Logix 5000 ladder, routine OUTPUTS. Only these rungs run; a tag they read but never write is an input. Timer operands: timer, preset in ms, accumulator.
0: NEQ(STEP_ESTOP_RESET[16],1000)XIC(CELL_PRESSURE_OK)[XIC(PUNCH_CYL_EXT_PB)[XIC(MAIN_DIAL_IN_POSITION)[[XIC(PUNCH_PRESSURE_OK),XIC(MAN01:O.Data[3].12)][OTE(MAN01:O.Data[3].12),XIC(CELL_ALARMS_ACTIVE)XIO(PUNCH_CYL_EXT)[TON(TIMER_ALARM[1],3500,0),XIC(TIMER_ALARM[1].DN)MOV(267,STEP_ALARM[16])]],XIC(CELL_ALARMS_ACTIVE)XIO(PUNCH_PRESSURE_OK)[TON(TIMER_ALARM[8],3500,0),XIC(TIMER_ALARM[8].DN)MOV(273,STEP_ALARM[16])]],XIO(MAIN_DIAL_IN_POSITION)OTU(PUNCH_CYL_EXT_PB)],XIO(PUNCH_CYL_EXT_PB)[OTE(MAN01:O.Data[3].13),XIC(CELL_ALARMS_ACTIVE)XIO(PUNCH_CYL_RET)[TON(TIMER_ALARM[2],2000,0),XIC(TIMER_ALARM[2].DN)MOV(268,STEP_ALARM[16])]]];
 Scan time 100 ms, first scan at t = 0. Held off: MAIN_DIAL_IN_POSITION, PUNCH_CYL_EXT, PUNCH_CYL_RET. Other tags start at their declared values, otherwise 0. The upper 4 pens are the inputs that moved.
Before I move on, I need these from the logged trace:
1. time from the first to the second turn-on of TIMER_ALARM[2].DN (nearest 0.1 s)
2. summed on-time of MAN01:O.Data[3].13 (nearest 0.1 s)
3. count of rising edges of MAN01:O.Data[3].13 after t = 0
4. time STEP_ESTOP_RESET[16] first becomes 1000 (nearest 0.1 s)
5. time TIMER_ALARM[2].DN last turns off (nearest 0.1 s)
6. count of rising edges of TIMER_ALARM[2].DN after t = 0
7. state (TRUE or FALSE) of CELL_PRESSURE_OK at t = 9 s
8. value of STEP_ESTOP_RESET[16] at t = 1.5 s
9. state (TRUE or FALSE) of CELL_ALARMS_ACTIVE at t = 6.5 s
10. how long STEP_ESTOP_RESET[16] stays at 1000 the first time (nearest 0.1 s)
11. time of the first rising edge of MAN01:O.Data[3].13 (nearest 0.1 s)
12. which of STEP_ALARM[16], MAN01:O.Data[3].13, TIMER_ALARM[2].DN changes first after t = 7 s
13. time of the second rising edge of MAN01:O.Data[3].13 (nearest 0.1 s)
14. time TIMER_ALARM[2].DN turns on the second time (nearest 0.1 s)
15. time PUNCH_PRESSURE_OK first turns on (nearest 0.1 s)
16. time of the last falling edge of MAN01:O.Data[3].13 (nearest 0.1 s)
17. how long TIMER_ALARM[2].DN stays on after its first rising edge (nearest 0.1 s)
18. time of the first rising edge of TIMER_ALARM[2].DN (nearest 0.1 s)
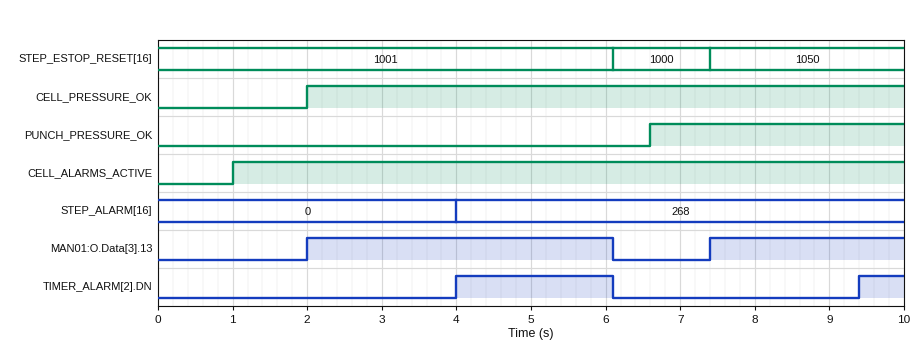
5.4 s
6.7 s
2
6.1 s
6.1 s
2
TRUE
1001
TRUE
1.3 s
2.0 s
MAN01:O.Data[3].13
7.4 s
9.4 s
6.6 s
6.1 s
2.1 s
4.0 s
